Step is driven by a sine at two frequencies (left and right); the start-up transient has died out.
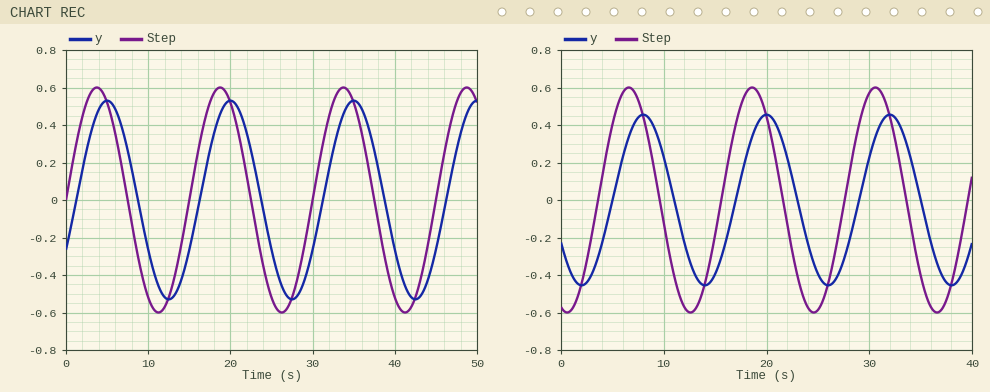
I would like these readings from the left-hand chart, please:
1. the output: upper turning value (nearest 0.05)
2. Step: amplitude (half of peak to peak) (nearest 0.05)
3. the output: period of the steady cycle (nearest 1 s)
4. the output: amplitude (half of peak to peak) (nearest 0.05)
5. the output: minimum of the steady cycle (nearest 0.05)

0.55
0.60
15 s
0.55
-0.55
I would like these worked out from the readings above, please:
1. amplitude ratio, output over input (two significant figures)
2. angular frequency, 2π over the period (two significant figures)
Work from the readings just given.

0.92
0.42 rad/s
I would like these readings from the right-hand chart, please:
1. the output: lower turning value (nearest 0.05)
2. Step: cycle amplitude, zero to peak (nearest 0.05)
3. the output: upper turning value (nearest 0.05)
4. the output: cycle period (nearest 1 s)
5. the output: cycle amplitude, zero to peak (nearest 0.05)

-0.45
0.60
0.45
12 s
0.45
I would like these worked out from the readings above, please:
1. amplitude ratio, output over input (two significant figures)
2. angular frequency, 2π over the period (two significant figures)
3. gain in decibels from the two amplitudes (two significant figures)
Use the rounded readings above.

0.75
0.52 rad/s
-2.5 dB
